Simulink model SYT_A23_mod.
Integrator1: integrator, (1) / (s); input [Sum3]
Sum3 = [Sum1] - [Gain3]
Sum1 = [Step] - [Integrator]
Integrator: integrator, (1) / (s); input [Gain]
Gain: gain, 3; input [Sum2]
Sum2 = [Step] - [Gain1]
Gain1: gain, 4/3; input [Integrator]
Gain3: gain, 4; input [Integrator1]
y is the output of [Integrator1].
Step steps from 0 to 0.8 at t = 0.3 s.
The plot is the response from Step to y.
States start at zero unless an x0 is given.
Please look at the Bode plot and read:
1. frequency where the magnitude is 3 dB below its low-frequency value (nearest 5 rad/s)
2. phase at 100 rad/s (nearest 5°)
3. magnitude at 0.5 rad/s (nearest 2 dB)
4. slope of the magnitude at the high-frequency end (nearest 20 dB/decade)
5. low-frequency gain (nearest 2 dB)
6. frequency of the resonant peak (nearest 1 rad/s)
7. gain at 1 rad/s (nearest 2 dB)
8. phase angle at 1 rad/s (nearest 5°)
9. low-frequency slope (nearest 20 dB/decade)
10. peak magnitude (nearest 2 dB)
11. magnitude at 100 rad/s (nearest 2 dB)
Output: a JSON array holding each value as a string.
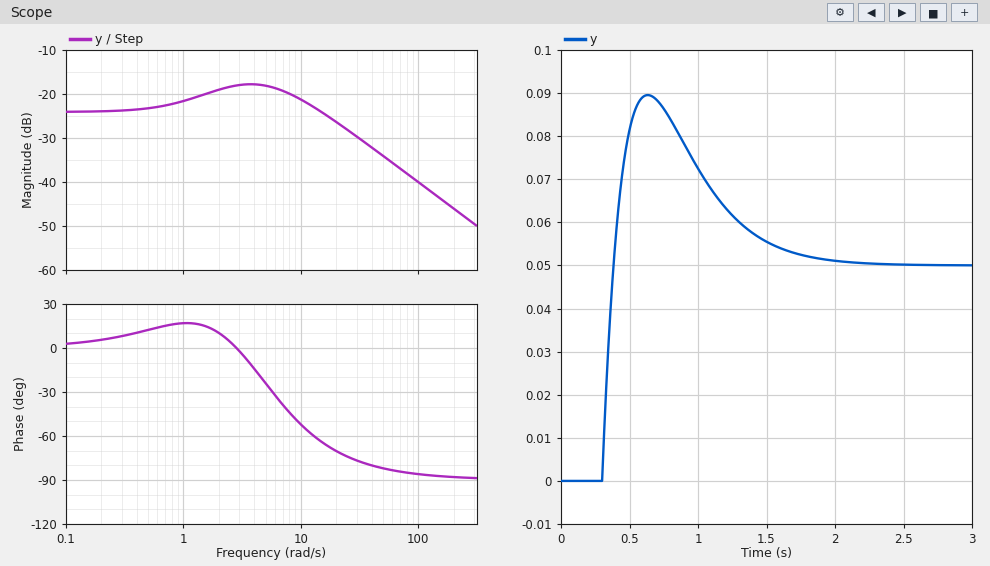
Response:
["20 rad/s", "-85°", "-24 dB", "-20 dB/decade", "-24 dB", "4 rad/s", "-22 dB", "15°", "0 dB/decade", "-18 dB", "-40 dB"]
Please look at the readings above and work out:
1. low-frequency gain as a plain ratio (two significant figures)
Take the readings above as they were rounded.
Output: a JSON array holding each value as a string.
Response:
["0.063"]
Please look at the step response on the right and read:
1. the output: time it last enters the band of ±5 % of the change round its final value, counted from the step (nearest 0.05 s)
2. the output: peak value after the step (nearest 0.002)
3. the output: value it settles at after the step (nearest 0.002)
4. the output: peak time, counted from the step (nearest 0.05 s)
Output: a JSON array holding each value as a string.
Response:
["1.45 s", "0.090", "0.050", "0.35 s"]
